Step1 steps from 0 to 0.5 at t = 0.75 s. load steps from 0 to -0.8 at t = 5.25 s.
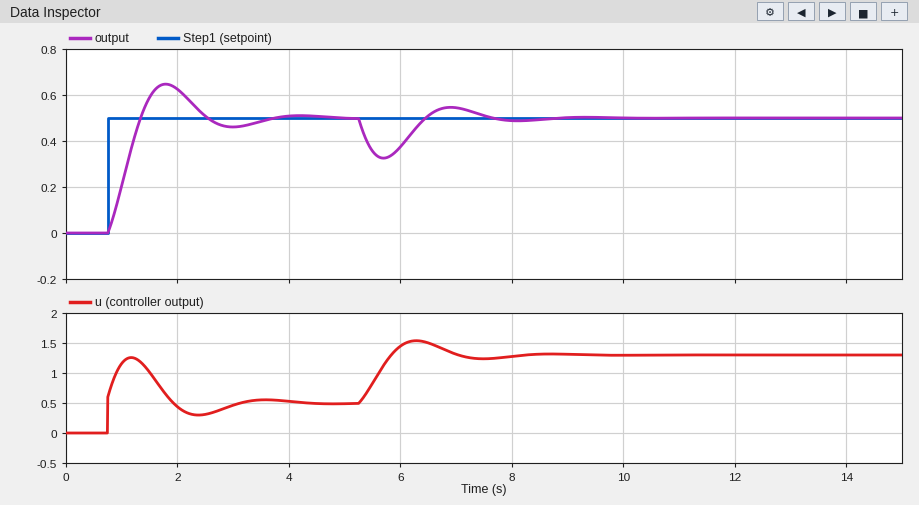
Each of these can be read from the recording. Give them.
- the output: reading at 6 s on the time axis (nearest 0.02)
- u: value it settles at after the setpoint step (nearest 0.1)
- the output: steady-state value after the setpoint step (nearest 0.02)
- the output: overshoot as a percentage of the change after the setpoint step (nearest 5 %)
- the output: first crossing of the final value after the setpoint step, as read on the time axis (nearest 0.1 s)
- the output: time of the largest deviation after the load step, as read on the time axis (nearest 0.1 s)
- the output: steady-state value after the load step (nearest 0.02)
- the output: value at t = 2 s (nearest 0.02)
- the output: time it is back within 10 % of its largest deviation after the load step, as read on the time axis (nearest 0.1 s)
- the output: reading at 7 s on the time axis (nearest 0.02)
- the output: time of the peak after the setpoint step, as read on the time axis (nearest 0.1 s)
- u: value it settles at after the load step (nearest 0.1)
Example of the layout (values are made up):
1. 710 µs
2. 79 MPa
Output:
1. 0.38
2. 0.5
3. 0.50
4. 30 %
5. 1.3 s
6. 5.7 s
7. 0.50
8. 0.62
9. 7.4 s
10. 0.54
11. 1.8 s
12. 1.3
